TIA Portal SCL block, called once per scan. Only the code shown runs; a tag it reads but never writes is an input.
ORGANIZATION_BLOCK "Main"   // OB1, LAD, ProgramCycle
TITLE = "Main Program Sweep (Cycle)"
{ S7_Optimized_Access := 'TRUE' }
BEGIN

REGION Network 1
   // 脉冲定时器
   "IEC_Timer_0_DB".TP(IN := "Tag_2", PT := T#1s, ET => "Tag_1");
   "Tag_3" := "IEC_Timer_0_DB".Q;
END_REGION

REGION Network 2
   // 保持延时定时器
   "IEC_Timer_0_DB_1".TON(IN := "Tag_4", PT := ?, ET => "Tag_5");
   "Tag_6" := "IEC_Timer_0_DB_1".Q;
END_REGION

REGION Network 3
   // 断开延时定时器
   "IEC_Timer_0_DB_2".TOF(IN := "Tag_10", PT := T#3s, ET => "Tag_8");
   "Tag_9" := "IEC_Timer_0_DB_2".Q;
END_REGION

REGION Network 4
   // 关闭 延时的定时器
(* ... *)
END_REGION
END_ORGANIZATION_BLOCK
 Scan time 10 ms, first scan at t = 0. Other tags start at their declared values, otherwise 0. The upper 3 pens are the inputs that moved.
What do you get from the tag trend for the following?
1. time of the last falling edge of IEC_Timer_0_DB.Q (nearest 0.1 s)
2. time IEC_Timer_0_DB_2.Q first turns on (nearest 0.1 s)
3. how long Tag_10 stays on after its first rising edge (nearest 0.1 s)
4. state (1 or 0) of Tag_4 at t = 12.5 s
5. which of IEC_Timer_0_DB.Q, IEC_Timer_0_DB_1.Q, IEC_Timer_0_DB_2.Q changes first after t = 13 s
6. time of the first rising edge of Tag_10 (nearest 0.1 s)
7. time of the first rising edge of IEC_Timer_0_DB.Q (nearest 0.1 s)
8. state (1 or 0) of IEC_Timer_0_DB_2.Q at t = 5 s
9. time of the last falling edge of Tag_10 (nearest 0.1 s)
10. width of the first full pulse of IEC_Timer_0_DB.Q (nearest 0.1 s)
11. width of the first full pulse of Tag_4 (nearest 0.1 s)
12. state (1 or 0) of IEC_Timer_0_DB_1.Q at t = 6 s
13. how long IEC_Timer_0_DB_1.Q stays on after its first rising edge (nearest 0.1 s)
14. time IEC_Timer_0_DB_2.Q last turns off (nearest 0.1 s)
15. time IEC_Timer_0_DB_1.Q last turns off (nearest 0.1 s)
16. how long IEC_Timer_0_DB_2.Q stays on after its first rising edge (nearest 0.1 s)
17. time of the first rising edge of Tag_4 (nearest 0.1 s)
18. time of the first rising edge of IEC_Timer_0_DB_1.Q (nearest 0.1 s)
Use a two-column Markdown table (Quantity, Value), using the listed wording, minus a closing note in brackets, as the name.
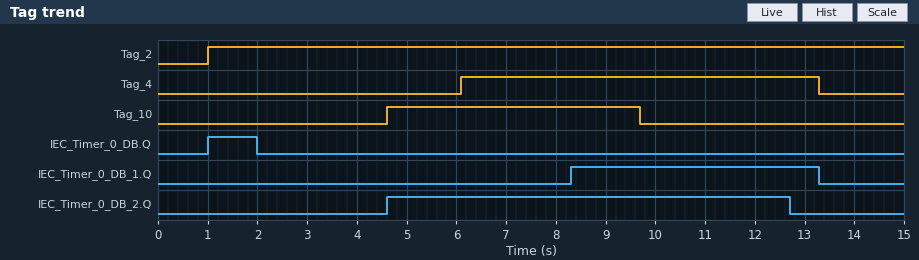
| Quantity | Value |
|---|---|
| time of the last falling edge of IEC_Timer_0_DB.Q | 2.0 s |
| time IEC_Timer_0_DB_2.Q first turns on | 4.6 s |
| how long Tag_10 stays on after its first rising edge | 5.1 s |
| state (1 or 0) of Tag_4 at t = 12.5 s | 1 |
| which of IEC_Timer_0_DB.Q, IEC_Timer_0_DB_1.Q, IEC_Timer_0_DB_2.Q changes first after t = 13 s | IEC_Timer_0_DB_1.Q |
| time of the first rising edge of Tag_10 | 4.6 s |
| time of the first rising edge of IEC_Timer_0_DB.Q | 1.0 s |
| state (1 or 0) of IEC_Timer_0_DB_2.Q at t = 5 s | 1 |
| time of the last falling edge of Tag_10 | 9.7 s |
| width of the first full pulse of IEC_Timer_0_DB.Q | 1.0 s |
| width of the first full pulse of Tag_4 | 7.2 s |
| state (1 or 0) of IEC_Timer_0_DB_1.Q at t = 6 s | 0 |
| how long IEC_Timer_0_DB_1.Q stays on after its first rising edge | 5.0 s |
| time IEC_Timer_0_DB_2.Q last turns off | 12.7 s |
| time IEC_Timer_0_DB_1.Q last turns off | 13.3 s |
| how long IEC_Timer_0_DB_2.Q stays on after its first rising edge | 8.1 s |
| time of the first rising edge of Tag_4 | 6.1 s |
| time of the first rising edge of IEC_Timer_0_DB_1.Q | 8.3 s |
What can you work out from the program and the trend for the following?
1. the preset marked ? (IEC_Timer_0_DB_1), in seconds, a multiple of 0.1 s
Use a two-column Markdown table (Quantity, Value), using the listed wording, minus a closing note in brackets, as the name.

| Quantity | Value |
|---|---|
| the preset marked ? (IEC_Timer_0_DB_1), in seconds, a multiple of 0.1 s | 2.2 s |
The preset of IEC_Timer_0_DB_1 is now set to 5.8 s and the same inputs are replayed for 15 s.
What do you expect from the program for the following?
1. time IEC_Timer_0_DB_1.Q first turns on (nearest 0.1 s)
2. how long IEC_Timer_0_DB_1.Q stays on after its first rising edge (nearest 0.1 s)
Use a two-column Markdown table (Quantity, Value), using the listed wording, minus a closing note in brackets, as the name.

| Quantity | Value |
|---|---|
| time IEC_Timer_0_DB_1.Q first turns on | 11.9 s |
| how long IEC_Timer_0_DB_1.Q stays on after its first rising edge | 1.4 s |
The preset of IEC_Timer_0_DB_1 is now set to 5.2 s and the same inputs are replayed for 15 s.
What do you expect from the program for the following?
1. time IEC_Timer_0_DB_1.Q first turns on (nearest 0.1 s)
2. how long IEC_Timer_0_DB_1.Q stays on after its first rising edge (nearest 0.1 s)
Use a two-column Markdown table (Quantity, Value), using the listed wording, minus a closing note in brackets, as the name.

| Quantity | Value |
|---|---|
| time IEC_Timer_0_DB_1.Q first turns on | 11.3 s |
| how long IEC_Timer_0_DB_1.Q stays on after its first rising edge | 2.0 s |
